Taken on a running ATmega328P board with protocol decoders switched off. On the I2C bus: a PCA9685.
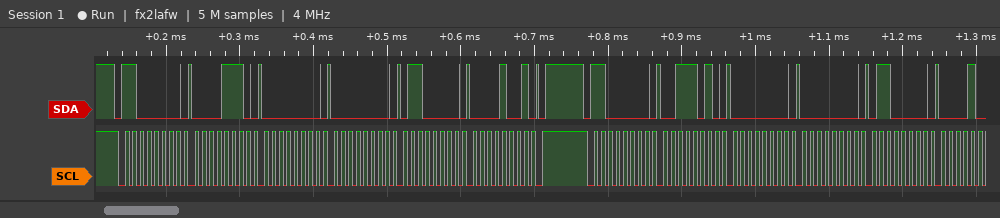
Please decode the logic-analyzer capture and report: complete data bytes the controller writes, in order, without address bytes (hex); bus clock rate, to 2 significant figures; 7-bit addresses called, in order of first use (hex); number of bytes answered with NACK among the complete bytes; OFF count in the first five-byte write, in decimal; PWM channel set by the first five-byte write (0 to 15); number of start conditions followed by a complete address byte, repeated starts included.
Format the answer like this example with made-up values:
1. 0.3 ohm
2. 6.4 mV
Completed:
1. 0E 00 00 60 09 3A 00 00 60
2. 100 kHz
3. 0x60
4. 0
5. 2400
6. 2
7. 2
